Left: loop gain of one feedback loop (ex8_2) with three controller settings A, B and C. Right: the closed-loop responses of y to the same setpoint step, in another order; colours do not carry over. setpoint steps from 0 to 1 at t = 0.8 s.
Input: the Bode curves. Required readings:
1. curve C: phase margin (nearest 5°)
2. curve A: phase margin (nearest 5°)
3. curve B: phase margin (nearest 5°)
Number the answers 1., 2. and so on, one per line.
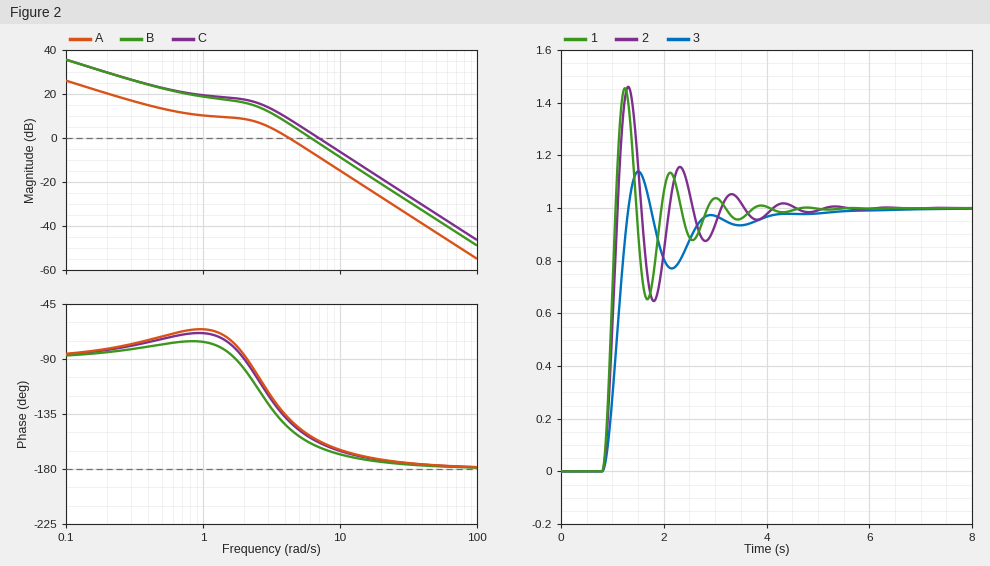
1. 20°
2. 40°
3. 20°
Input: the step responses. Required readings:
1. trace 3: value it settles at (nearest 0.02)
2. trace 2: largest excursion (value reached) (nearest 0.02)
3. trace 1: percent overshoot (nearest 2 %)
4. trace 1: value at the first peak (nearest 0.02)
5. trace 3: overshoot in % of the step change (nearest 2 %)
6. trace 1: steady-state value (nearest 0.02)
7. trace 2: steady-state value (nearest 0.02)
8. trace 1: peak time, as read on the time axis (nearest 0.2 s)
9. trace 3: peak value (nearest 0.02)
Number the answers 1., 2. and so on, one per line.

1. 1.00
2. 1.46
3. 46 %
4. 1.46
5. 14 %
6. 1.00
7. 1.00
8. 1.2 s
9. 1.14
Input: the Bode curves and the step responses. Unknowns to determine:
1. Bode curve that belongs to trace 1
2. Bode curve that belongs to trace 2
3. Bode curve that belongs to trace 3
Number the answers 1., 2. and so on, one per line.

1. C
2. B
3. A
